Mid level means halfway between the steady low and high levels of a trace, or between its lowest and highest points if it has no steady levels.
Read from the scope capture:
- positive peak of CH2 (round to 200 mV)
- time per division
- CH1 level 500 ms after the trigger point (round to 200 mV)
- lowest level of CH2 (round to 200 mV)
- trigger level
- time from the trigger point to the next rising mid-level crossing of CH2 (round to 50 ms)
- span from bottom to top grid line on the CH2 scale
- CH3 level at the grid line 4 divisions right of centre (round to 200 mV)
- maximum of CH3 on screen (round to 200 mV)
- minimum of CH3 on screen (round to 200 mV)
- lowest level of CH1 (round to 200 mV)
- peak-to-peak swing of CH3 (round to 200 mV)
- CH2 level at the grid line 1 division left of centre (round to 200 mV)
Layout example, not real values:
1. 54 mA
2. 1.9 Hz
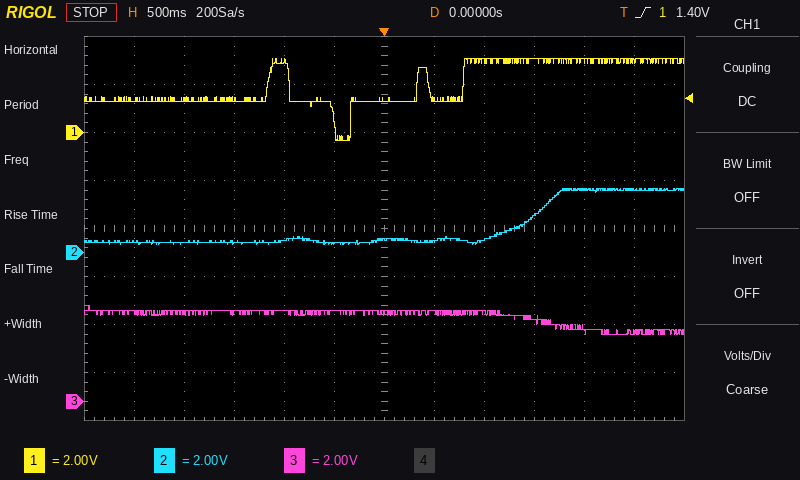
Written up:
1. 2.6 V
2. 500 ms
3. 1.4 V
4. 400 mV
5. 1.40 V
6. 1.50 s
7. 16 V
8. 3.0 V
9. 4.0 V
10. 2.8 V
11. -400 mV
12. 1.2 V
13. 400 mV
